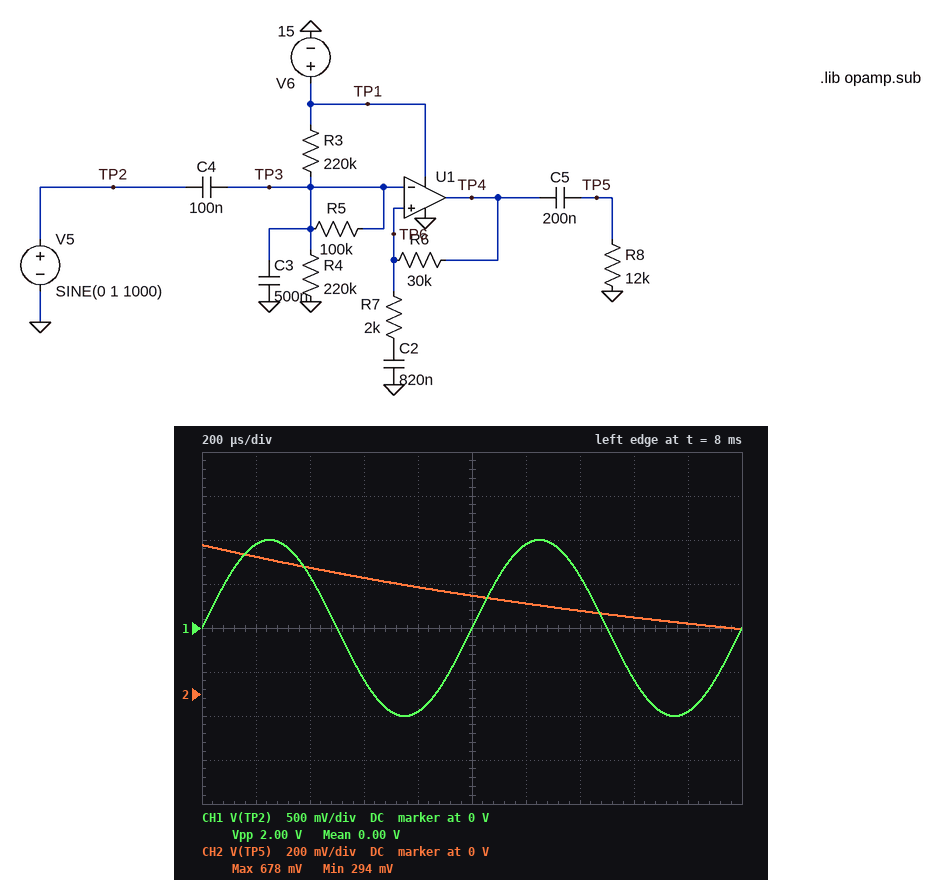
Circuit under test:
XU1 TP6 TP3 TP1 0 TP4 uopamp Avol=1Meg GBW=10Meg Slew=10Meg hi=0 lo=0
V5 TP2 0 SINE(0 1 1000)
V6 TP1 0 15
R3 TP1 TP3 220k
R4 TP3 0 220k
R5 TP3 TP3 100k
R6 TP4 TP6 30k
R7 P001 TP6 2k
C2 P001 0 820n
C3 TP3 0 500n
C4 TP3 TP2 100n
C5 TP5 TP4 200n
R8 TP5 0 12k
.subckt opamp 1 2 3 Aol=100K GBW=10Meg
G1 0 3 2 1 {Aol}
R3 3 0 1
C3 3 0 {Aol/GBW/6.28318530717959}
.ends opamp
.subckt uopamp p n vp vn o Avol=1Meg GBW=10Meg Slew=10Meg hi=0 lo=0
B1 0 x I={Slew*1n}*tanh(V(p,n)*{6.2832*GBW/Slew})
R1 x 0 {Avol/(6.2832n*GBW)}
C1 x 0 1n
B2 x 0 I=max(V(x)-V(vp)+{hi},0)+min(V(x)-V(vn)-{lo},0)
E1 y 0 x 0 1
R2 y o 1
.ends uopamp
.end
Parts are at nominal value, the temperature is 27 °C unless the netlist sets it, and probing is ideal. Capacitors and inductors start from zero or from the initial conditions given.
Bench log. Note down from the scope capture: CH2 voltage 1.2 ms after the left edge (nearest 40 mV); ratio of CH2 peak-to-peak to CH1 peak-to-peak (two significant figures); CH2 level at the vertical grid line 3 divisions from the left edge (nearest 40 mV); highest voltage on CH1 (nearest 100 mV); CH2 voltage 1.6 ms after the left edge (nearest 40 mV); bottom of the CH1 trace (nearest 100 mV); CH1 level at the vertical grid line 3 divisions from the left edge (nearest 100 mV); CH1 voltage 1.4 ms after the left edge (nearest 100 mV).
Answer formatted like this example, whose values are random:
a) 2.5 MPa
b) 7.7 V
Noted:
a) 400 mV
b) 0.19
c) 520 mV
d) 1.0 V
e) 360 mV
f) -1.0 V
g) -600 mV
h) 600 mV
